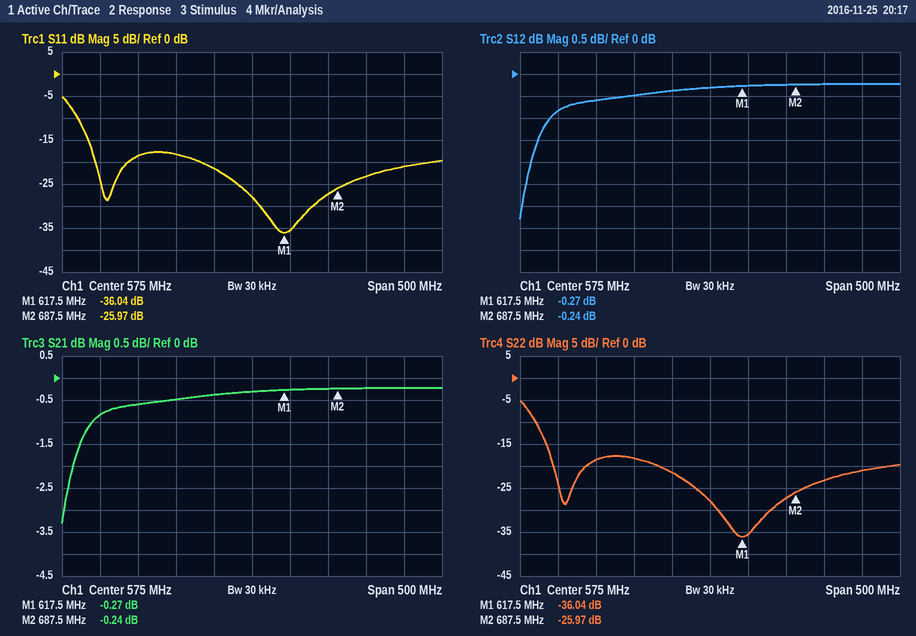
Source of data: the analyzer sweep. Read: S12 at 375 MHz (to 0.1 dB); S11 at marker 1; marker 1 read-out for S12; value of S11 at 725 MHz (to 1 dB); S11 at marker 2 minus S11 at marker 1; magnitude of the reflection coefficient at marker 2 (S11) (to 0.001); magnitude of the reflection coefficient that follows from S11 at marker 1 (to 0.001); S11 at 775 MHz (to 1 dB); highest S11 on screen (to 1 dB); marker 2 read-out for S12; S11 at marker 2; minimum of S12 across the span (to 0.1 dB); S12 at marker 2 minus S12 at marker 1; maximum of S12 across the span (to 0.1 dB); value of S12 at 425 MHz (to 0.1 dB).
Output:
-0.8 dB
-36.04 dB
-0.27 dB
-23 dB
10.07 dB
0.050
0.016
-21 dB
-5 dB
-0.24 dB
-25.97 dB
-3.3 dB
0.03 dB
-0.2 dB
-0.6 dB
